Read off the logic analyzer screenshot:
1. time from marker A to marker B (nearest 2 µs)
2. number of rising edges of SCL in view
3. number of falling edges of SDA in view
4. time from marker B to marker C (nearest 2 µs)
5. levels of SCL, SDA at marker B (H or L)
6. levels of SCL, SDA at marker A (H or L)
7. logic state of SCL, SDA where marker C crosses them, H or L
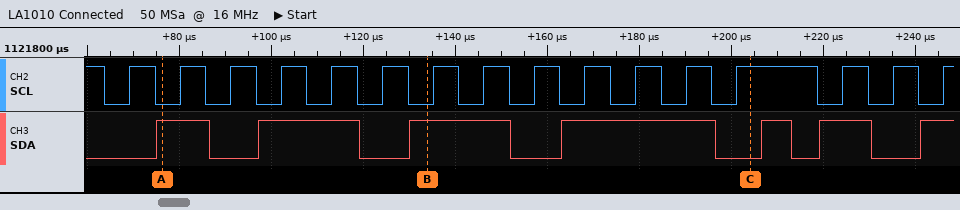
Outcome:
58 µs
16
6
70 µs
SCL=L, SDA=H
SCL=L, SDA=H
SCL=H, SDA=L
